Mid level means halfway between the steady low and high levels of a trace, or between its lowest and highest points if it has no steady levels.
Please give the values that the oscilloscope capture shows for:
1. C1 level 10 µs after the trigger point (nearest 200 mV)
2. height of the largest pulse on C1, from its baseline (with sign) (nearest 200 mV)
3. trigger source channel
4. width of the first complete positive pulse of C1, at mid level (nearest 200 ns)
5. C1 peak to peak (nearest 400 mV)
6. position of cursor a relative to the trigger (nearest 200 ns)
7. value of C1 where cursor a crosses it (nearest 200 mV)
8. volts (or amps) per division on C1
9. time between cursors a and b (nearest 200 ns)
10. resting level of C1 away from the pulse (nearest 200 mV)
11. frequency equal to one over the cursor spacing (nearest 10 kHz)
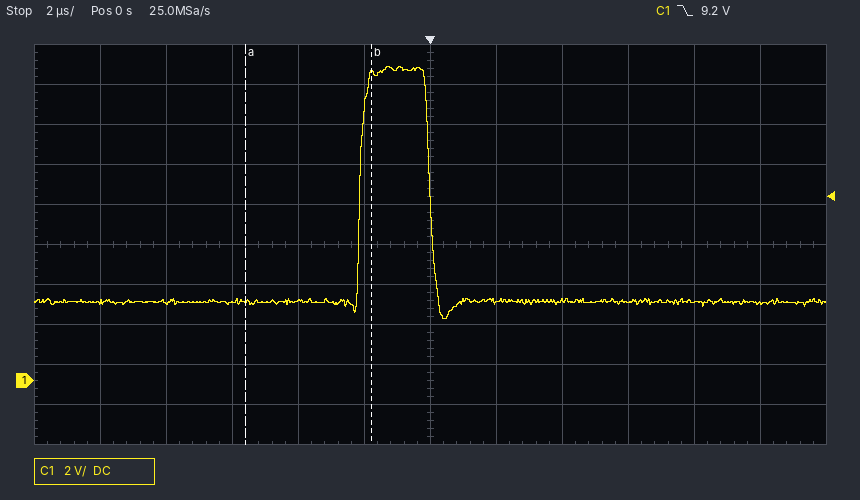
3.8 V
+11.8 V
C1
2.2 µs
12.8 V
-5.6 µs
4.0 V
2 V
3.8 µs
4.0 V
260 kHz
